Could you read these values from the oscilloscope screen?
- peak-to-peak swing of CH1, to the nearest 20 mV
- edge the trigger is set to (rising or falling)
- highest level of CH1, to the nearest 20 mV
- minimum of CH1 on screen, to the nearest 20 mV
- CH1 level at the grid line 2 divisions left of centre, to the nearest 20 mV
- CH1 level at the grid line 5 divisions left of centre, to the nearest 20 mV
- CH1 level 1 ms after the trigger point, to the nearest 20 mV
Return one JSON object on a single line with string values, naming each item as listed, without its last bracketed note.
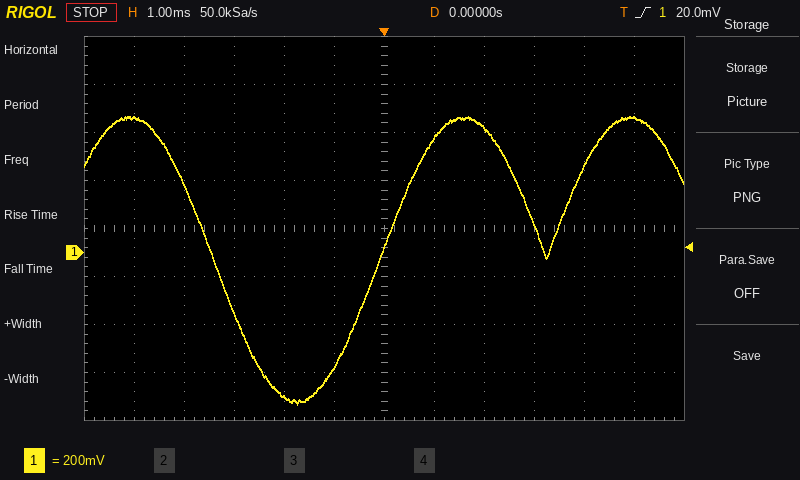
{"peak-to-peak swing of CH1, to the nearest 20 mV": "1.20 V", "edge the trigger is set to": "rising", "highest level of CH1, to the nearest 20 mV": "560 mV", "minimum of CH1 on screen, to the nearest 20 mV": "-640 mV", "CH1 level at the grid line 2 divisions left of centre, to the nearest 20 mV": "-600 mV", "CH1 level at the grid line 5 divisions left of centre, to the nearest 20 mV": "560 mV", "CH1 level 1 ms after the trigger point, to the nearest 20 mV": "480 mV"}
